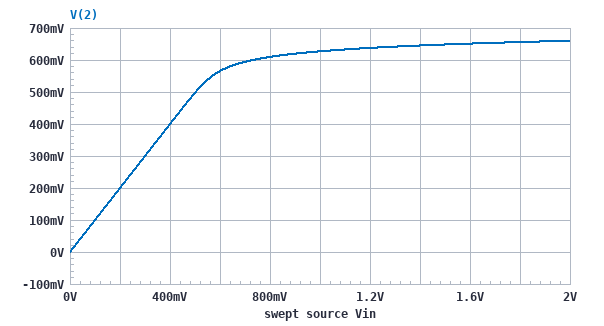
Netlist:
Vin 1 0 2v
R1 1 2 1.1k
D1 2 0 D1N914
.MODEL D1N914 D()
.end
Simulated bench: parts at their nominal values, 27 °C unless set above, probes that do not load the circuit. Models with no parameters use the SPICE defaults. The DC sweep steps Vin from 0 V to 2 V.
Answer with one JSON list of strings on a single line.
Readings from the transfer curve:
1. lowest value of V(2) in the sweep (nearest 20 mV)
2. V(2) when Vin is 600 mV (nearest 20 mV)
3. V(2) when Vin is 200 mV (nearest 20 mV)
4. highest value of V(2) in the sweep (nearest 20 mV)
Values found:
["0 V", "560 mV", "200 mV", "660 mV"]
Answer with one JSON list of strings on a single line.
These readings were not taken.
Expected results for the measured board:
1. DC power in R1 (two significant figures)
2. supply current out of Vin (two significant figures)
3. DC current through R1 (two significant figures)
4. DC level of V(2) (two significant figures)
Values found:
["1.6 mW", "1.2 mA", "1.2 mA", "660 mV"]
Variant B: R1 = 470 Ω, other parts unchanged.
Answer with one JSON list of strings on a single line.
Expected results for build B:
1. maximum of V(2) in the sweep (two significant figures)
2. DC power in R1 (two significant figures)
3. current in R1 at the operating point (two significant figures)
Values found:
["680 mV", "3.7 mW", "2.8 mA"]
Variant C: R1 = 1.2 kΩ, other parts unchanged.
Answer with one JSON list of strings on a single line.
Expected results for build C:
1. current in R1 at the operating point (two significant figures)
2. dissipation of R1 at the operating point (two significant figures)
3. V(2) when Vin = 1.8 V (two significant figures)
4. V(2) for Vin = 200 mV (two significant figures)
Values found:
["1.1 mA", "1.5 mW", "650 mV", "200 mV"]
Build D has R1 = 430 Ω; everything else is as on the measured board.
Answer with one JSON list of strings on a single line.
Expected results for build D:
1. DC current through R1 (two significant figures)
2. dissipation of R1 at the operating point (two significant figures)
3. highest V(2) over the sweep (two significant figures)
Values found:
["3.1 mA", "4.0 mW", "680 mV"]
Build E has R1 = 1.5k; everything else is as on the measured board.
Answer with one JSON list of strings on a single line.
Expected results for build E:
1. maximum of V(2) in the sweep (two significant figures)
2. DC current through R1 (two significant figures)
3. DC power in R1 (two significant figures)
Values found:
["650 mV", "900 µA", "1.2 mW"]
